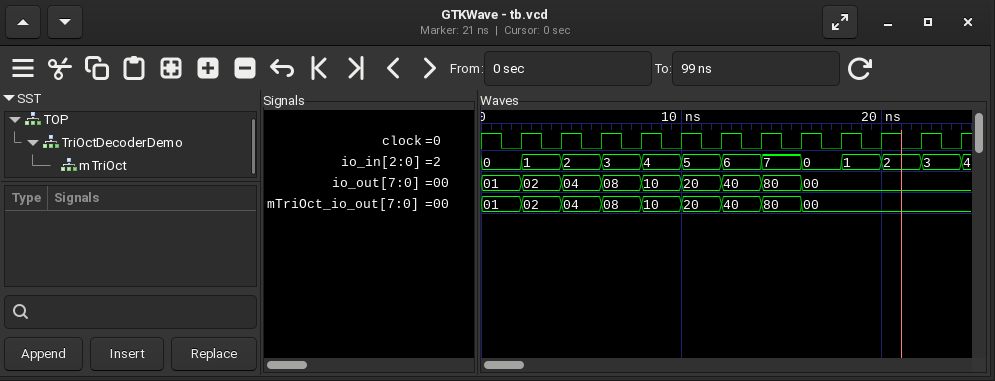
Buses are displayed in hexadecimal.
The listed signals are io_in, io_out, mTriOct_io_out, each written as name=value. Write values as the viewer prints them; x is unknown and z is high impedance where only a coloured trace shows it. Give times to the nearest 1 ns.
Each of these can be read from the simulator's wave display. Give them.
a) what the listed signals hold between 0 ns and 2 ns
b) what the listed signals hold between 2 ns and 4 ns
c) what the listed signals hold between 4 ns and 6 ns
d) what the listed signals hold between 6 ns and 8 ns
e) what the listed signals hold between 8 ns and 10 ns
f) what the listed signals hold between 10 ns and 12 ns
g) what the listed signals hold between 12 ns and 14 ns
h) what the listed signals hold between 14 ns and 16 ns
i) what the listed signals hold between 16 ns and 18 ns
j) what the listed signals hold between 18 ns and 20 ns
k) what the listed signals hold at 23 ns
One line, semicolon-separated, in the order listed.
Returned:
io_in=0, io_out=01, mTriOct_io_out=01; io_in=1, io_out=02, mTriOct_io_out=02; io_in=2, io_out=04, mTriOct_io_out=04; io_in=3, io_out=08, mTriOct_io_out=08; io_in=4, io_out=10, mTriOct_io_out=10; io_in=5, io_out=20, mTriOct_io_out=20; io_in=6, io_out=40, mTriOct_io_out=40; io_in=7, io_out=80, mTriOct_io_out=80; io_in=0, io_out=00, mTriOct_io_out=00; io_in=1, io_out=00, mTriOct_io_out=00; io_in=3, io_out=00, mTriOct_io_out=00
